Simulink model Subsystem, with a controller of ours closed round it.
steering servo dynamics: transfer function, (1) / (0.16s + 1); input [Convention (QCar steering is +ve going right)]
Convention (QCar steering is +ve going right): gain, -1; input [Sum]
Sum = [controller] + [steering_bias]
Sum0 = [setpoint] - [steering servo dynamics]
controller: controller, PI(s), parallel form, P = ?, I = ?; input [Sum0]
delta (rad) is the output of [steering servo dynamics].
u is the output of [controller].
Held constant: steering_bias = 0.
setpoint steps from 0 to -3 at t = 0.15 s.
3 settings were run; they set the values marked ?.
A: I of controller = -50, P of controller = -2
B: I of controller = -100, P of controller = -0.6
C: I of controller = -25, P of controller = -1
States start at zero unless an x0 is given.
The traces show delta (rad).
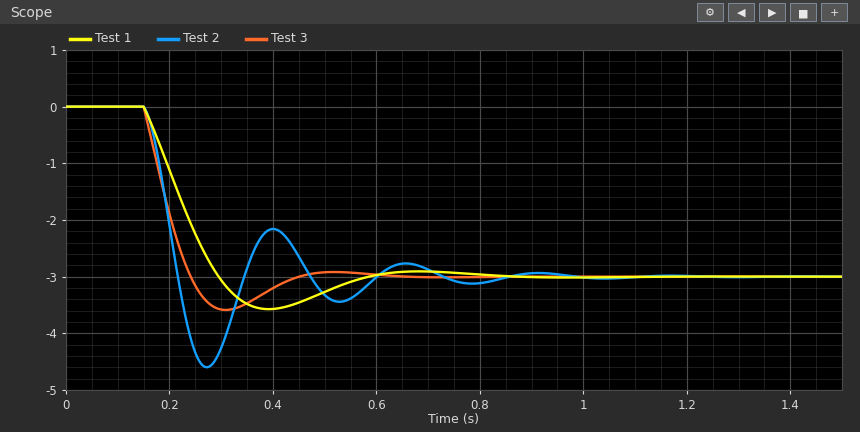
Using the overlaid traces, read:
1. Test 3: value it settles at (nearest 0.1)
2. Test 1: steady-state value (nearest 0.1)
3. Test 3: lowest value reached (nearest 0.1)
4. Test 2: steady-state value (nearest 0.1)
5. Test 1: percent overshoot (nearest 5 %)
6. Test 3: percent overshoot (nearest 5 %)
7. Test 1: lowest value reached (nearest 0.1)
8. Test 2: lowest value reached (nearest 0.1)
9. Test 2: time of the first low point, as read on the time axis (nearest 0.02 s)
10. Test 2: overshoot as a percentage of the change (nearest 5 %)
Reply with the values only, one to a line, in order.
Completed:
-3.0
-3.0
-3.6
-3.0
20 %
20 %
-3.6
-4.6
0.28 s
55 %
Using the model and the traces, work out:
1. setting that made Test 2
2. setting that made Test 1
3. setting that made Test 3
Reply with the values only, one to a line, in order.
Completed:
B
C
A
